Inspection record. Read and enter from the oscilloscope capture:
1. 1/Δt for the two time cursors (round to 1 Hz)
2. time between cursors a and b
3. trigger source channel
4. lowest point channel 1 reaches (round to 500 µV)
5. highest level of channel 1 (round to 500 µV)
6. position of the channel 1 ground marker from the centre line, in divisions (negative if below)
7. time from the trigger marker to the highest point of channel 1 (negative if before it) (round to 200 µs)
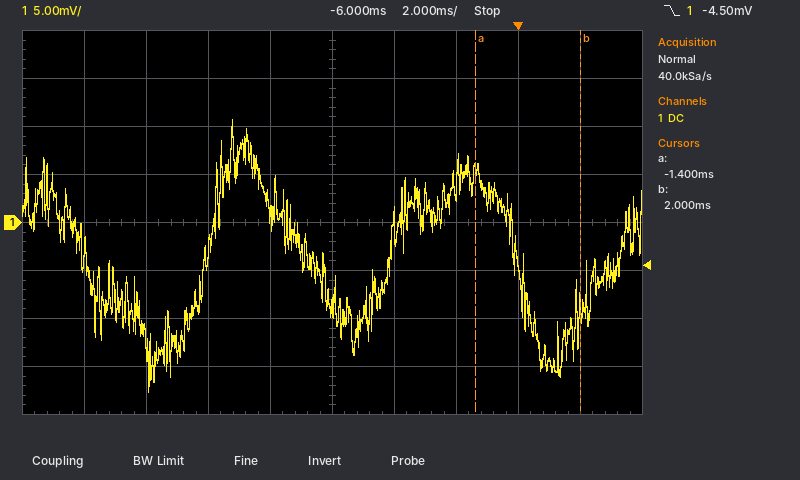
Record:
294 Hz
3.4 ms
channel 1
-17.5 mV
10.5 mV
0.0 div
-9.2 ms
